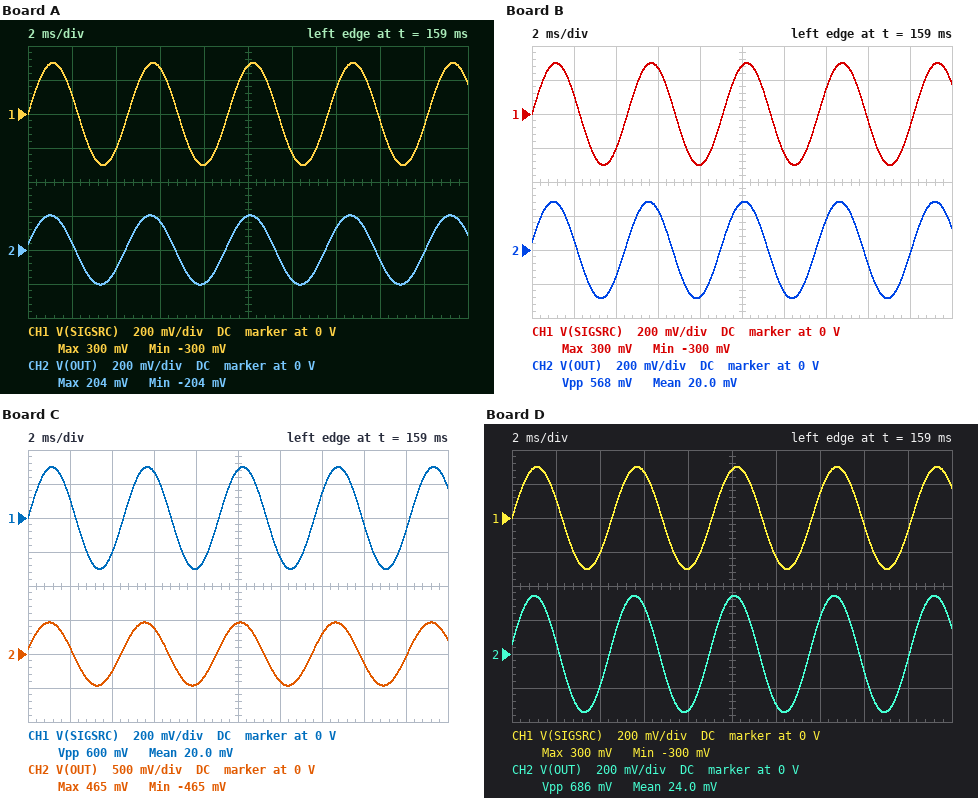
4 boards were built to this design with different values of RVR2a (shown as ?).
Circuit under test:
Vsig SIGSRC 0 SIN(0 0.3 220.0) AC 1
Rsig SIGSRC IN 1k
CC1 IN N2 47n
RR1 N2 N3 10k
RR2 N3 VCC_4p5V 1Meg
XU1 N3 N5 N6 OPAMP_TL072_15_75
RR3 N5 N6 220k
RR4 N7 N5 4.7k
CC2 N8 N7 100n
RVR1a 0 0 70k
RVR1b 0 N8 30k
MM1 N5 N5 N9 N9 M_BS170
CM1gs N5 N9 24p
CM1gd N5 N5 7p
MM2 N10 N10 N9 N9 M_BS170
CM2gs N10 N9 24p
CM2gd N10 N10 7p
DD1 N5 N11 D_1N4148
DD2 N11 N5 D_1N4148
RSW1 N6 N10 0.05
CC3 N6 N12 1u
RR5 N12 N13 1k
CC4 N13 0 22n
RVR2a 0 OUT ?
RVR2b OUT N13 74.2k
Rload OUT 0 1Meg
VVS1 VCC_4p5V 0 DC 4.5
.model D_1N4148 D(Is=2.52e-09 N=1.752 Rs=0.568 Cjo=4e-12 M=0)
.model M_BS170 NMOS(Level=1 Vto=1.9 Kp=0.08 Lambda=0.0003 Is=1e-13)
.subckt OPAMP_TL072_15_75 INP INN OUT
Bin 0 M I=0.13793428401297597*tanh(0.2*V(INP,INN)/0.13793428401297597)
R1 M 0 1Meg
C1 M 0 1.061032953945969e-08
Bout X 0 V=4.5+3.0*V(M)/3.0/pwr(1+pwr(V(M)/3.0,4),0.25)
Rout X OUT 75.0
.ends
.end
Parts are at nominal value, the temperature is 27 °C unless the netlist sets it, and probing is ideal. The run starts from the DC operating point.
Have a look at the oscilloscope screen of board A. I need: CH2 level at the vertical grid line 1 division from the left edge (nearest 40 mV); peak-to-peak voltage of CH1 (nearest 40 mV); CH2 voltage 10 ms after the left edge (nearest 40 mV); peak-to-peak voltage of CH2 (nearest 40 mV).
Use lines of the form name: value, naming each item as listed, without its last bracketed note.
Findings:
CH2 level at the vertical grid line 1 division from the left edge: 40 mV
peak-to-peak voltage of CH1: 600 mV
CH2 voltage 10 ms after the left edge: 200 mV
peak-to-peak voltage of CH2: 400 mV
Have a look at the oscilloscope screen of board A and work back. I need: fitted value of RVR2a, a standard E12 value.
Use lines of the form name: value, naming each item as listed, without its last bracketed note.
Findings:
fitted value of RVR2a, a standard E12 value: 8.2 kΩ
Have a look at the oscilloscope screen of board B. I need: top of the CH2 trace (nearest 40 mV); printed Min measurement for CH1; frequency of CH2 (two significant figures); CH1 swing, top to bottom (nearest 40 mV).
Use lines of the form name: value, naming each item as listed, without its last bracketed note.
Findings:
top of the CH2 trace: 280 mV
printed Min measurement for CH1: -300 mV
frequency of CH2: 220 Hz
CH1 swing, top to bottom: 600 mV
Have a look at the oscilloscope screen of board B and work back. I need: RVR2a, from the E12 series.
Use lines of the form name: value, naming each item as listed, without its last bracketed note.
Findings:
RVR2a, from the E12 series: 12 kΩ
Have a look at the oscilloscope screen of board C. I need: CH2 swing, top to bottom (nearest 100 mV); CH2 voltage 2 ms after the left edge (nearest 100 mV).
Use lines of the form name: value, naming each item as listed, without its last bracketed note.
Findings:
CH2 swing, top to bottom: 900 mV
CH2 voltage 2 ms after the left edge: 100 mV
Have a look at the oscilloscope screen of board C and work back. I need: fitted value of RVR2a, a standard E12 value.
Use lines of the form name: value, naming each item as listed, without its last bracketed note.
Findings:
fitted value of RVR2a, a standard E12 value: 22 kΩ
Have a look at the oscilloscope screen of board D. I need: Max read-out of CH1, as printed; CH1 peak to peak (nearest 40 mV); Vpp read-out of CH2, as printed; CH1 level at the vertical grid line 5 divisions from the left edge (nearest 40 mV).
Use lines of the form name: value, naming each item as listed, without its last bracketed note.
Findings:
Max read-out of CH1, as printed: 300 mV
CH1 peak to peak: 600 mV
Vpp read-out of CH2, as printed: 686 mV
CH1 level at the vertical grid line 5 divisions from the left edge: 280 mV
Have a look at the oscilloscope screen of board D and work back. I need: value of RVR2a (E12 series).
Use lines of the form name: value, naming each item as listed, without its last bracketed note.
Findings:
value of RVR2a: 15 kΩ
